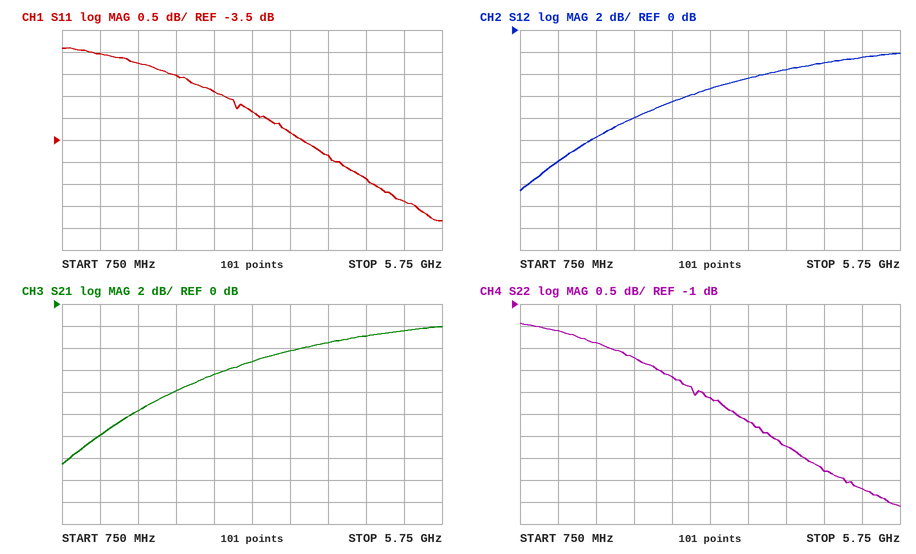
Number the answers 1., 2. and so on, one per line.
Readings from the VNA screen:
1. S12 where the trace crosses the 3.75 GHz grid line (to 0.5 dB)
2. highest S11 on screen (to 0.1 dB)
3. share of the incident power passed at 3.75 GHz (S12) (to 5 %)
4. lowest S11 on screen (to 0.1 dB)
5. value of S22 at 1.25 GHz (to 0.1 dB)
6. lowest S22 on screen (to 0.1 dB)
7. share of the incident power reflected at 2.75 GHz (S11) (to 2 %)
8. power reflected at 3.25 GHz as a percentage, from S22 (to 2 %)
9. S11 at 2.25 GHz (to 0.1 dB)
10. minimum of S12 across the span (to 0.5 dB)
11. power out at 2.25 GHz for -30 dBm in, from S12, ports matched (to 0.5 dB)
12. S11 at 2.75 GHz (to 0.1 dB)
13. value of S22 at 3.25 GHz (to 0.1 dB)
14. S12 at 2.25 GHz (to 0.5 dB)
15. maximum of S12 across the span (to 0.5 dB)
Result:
1. -4.5 dB
2. -1.4 dB
3. 35 %
4. -5.3 dB
5. -1.6 dB
6. -5.6 dB
7. 58 %
8. 48 %
9. -2.0 dB
10. -14.5 dB
11. -38.0 dBm
12. -2.4 dB
13. -3.1 dB
14. -8.0 dB
15. -2.0 dB
